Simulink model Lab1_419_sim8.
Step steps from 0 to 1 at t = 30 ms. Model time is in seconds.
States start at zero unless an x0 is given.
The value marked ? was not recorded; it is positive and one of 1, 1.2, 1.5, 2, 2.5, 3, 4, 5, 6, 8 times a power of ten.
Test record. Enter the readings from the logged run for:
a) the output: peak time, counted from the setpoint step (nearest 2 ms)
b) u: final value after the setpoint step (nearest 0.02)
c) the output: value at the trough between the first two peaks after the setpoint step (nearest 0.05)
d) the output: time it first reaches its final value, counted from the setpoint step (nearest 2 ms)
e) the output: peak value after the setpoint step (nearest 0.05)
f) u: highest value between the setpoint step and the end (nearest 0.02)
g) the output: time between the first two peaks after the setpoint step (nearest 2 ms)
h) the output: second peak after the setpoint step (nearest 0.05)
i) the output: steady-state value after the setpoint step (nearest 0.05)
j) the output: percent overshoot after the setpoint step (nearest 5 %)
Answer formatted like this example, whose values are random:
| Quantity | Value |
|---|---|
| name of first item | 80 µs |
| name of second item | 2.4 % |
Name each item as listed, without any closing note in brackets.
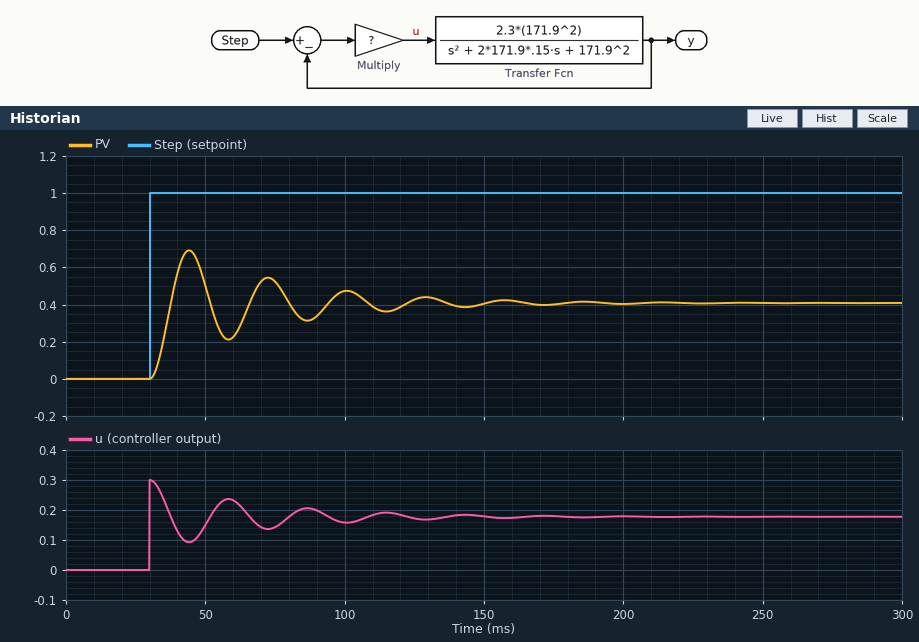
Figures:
| Quantity | Value |
|---|---|
| the output: peak time, counted from the setpoint step | 14 ms |
| u: final value after the setpoint step | 0.18 |
| the output: value at the trough between the first two peaks after the setpoint step | 0.20 |
| the output: time it first reaches its final value, counted from the setpoint step | 8 ms |
| the output: peak value after the setpoint step | 0.70 |
| u: highest value between the setpoint step and the end | 0.30 |
| the output: time between the first two peaks after the setpoint step | 28 ms |
| the output: second peak after the setpoint step | 0.55 |
| the output: steady-state value after the setpoint step | 0.40 |
| the output: percent overshoot after the setpoint step | 70 % |
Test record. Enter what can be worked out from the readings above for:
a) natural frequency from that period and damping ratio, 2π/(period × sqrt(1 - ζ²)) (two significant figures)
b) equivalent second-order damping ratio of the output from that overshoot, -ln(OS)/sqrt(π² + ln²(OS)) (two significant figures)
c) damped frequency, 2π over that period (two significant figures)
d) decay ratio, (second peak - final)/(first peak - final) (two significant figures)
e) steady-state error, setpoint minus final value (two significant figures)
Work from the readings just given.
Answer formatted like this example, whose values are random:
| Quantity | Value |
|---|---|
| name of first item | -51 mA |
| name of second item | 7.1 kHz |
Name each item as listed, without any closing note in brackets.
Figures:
| Quantity | Value |
|---|---|
| natural frequency from that period and damping ratio, 2π/(period × sqrt(1 - ζ²)) | 0.23 rad/ms |
| equivalent second-order damping ratio of the output from that overshoot, -ln(OS)/sqrt(π² + ln²(OS)) | 0.11 |
| damped frequency, 2π over that period | 0.22 rad/ms |
| decay ratio, (second peak - final)/(first peak - final) | 0.50 |
| steady-state error, setpoint minus final value | 0.60 |
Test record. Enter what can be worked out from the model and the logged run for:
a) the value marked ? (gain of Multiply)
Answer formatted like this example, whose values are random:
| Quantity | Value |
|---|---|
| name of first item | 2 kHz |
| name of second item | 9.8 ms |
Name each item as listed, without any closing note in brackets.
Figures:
| Quantity | Value |
|---|---|
| the value marked ? | 0.3 |
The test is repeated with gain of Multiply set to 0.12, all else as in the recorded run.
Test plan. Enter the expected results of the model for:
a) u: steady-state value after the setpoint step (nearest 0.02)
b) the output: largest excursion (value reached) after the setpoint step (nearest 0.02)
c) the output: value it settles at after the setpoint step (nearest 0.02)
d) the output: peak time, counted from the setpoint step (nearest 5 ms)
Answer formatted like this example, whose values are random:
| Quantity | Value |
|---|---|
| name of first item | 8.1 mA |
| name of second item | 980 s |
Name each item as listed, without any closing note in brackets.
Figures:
| Quantity | Value |
|---|---|
| u: steady-state value after the setpoint step | 0.10 |
| the output: largest excursion (value reached) after the setpoint step | 0.36 |
| the output: value it settles at after the setpoint step | 0.22 |
| the output: peak time, counted from the setpoint step | 15 ms |
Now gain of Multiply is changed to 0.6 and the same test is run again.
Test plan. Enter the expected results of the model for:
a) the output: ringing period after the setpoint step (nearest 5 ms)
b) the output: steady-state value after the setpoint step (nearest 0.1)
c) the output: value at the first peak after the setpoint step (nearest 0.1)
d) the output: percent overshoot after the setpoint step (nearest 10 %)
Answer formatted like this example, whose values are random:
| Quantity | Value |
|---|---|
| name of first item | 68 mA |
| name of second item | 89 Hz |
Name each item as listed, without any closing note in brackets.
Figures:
| Quantity | Value |
|---|---|
| the output: ringing period after the setpoint step | 25 ms |
| the output: steady-state value after the setpoint step | 0.6 |
| the output: value at the first peak after the setpoint step | 1.0 |
| the output: percent overshoot after the setpoint step | 70 % |
